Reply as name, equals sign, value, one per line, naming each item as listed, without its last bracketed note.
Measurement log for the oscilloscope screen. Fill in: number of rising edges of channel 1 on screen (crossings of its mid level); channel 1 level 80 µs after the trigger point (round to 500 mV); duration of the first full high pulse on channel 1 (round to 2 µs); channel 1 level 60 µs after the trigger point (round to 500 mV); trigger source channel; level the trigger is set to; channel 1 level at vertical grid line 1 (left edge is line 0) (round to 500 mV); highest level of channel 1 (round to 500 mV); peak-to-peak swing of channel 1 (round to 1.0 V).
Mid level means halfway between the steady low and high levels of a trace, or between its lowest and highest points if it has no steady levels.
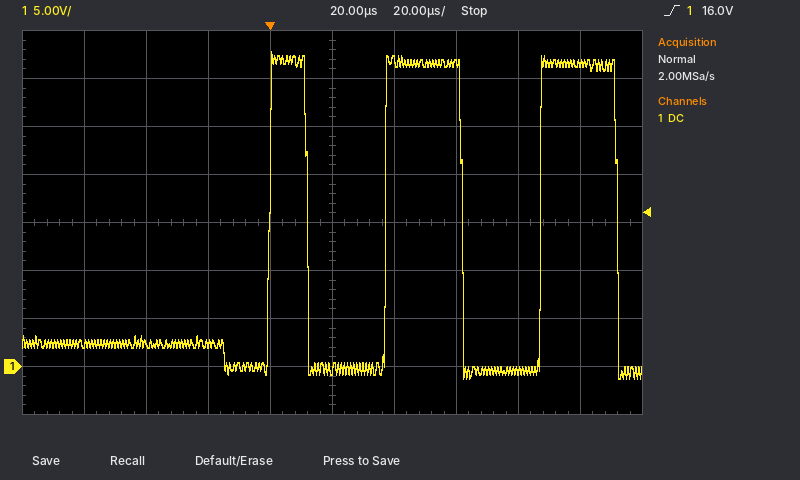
number of rising edges of channel 1 on screen = 3
channel 1 level 80 µs after the trigger point = -500 mV
duration of the first full high pulse on channel 1 = 12 µs
channel 1 level 60 µs after the trigger point = 31.5 V
trigger source channel = channel 1
level the trigger is set to = 16.0 V
channel 1 level at vertical grid line 1 (left edge is line 0) = 2.5 V
highest level of channel 1 = 33.0 V
peak-to-peak swing of channel 1 = 34.0 V
